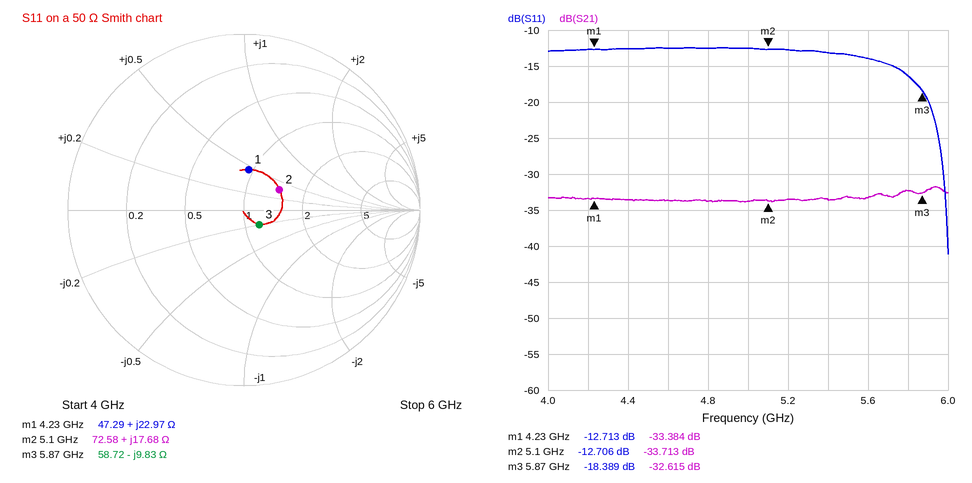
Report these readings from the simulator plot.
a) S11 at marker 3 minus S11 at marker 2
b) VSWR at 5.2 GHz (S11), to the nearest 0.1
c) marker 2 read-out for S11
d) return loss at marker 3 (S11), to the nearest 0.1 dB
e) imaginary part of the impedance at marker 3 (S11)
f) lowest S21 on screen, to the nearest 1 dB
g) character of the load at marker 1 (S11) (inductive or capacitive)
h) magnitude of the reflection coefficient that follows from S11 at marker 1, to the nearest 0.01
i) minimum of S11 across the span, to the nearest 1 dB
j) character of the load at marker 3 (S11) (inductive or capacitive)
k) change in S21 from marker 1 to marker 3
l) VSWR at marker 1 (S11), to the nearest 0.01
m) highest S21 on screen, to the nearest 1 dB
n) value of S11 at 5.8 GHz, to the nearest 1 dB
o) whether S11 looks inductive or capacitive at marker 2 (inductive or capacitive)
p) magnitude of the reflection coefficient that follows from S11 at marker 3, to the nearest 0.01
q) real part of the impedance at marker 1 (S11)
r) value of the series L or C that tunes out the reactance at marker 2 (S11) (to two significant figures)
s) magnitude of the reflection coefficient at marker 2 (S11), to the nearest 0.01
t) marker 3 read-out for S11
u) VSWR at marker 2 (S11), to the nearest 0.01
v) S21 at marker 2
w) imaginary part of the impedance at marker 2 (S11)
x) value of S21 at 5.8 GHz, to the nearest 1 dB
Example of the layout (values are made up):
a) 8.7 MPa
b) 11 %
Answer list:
a) -5.683 dB
b) 1.6
c) -12.706 dB
d) 18.4 dB
e) -9.83 Ω
f) -34 dB
g) inductive
h) 0.23
i) -41 dB
j) capacitive
k) 0.769 dB
l) 1.60
m) -32 dB
n) -16 dB
o) inductive
p) 0.12
q) 47.29 Ω
r) 1.8 pF
s) 0.23
t) -18.389 dB
u) 1.60
v) -33.713 dB
w) +17.68 Ω
x) -32 dB
